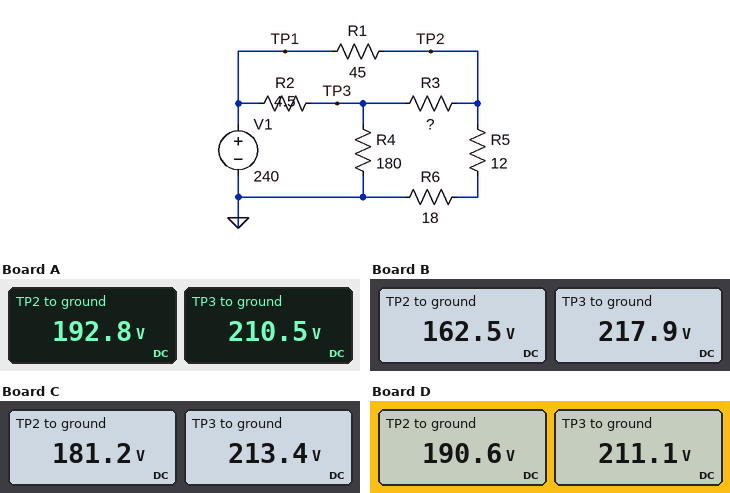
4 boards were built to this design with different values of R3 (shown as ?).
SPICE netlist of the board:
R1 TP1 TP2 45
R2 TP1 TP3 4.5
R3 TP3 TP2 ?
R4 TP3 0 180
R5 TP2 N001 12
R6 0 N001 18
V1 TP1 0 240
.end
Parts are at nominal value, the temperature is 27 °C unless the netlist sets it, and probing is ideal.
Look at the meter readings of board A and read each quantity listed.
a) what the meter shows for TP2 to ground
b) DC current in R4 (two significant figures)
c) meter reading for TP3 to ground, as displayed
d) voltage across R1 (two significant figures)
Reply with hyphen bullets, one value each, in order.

- 192.8 V
- 1.2 A
- 210.5 V
- 47 V
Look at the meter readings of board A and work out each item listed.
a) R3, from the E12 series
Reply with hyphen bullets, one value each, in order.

- 3.3 Ω
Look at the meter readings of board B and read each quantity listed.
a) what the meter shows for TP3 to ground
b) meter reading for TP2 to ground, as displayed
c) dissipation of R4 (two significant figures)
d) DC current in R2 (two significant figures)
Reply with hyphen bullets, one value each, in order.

- 217.9 V
- 162.5 V
- 260 W
- 4.9 A
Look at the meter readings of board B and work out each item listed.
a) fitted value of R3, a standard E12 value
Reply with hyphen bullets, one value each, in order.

- 15 Ω
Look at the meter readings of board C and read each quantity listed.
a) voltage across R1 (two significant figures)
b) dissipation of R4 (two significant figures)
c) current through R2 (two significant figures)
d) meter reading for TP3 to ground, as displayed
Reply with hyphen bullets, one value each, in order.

- 59 V
- 250 W
- 5.9 A
- 213.4 V
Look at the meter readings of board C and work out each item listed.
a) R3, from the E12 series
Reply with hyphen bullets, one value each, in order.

- 6.8 Ω
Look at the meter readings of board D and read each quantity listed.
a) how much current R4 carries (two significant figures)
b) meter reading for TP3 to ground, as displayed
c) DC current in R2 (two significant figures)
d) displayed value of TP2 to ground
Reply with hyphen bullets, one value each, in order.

- 1.2 A
- 211.1 V
- 6.4 A
- 190.6 V
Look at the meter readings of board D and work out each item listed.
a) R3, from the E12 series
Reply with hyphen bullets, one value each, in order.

- 3.9 Ω
